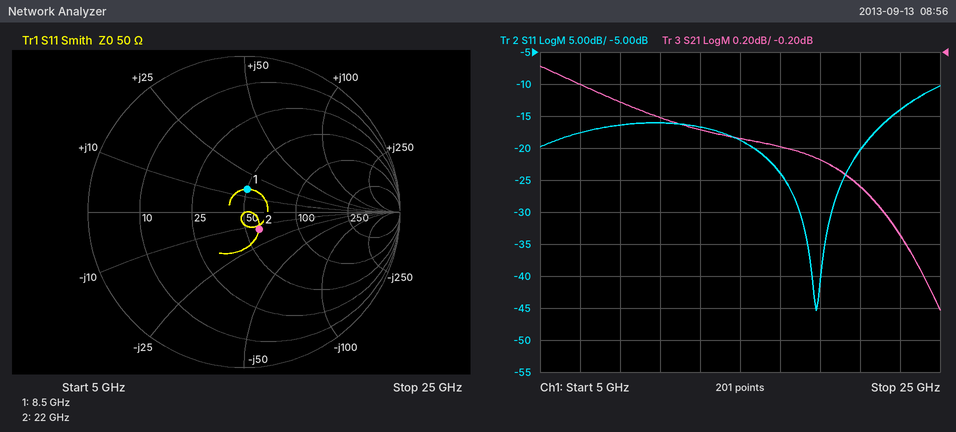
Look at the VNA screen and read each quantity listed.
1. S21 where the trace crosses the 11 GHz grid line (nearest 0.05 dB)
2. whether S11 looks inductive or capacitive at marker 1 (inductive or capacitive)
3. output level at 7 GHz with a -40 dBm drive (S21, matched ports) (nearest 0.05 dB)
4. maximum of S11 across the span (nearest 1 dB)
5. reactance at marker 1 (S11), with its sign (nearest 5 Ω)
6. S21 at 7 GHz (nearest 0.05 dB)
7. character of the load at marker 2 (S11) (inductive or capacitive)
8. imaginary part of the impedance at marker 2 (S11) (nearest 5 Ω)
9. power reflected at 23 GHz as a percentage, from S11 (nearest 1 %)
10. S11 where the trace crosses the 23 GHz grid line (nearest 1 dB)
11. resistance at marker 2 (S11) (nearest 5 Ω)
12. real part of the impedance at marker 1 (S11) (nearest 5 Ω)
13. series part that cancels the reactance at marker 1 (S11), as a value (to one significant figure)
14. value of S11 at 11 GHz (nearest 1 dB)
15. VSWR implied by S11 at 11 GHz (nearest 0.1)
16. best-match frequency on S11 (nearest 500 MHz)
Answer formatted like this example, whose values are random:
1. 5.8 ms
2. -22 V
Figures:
1. -0.60 dB
2. inductive
3. -40.40 dBm
4. -10 dB
5. +15 Ω
6. -0.40 dB
7. capacitive
8. -15 Ω
9. 4 %
10. -14 dB
11. 60 Ω
12. 50 Ω
13. 1 pF
14. -16 dB
15. 1.4
16. 19.0 GHz
